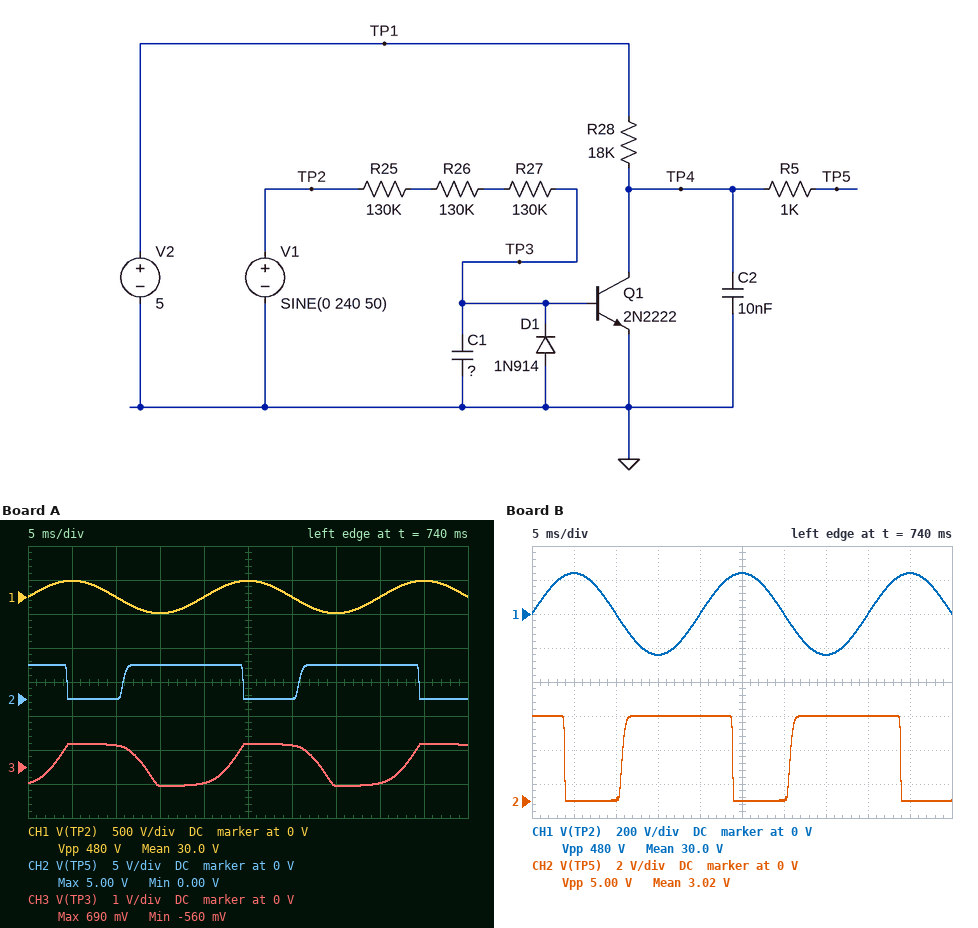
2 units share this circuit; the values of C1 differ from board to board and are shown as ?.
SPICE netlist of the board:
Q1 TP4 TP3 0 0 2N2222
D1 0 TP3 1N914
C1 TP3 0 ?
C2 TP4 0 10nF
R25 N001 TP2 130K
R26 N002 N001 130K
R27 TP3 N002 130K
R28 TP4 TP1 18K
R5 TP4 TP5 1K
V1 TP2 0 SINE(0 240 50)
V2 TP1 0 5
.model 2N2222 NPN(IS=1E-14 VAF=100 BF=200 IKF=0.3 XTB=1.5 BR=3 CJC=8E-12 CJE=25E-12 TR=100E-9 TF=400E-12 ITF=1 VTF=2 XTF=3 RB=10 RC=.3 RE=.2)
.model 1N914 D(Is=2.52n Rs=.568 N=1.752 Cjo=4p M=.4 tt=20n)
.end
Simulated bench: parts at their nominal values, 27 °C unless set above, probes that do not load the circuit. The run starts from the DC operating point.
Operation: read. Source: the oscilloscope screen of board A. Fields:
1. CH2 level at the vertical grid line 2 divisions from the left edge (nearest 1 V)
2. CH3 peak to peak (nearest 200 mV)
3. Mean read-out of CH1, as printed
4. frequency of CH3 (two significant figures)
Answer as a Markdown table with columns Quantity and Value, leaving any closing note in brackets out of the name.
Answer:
| Quantity | Value |
|---|---|
| CH2 level at the vertical grid line 2 divisions from the left edge | 0 V |
| CH3 peak to peak | 1.2 V |
| Mean read-out of CH1, as printed | 30.0 V |
| frequency of CH3 | 50 Hz |
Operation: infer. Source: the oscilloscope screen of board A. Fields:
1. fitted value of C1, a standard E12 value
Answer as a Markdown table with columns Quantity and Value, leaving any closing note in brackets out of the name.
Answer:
| Quantity | Value |
|---|---|
| fitted value of C1, a standard E12 value | 1.5 µF |
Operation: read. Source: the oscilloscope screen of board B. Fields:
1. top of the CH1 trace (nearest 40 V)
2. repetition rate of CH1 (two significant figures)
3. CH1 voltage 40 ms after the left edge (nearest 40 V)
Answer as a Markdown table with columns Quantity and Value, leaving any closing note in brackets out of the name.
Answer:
| Quantity | Value |
|---|---|
| top of the CH1 trace | 240 V |
| repetition rate of CH1 | 50 Hz |
| CH1 voltage 40 ms after the left edge | 0 V |
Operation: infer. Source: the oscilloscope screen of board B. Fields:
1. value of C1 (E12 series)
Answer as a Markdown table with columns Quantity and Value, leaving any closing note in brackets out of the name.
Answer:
| Quantity | Value |
|---|---|
| value of C1 | 1.2 µF |
